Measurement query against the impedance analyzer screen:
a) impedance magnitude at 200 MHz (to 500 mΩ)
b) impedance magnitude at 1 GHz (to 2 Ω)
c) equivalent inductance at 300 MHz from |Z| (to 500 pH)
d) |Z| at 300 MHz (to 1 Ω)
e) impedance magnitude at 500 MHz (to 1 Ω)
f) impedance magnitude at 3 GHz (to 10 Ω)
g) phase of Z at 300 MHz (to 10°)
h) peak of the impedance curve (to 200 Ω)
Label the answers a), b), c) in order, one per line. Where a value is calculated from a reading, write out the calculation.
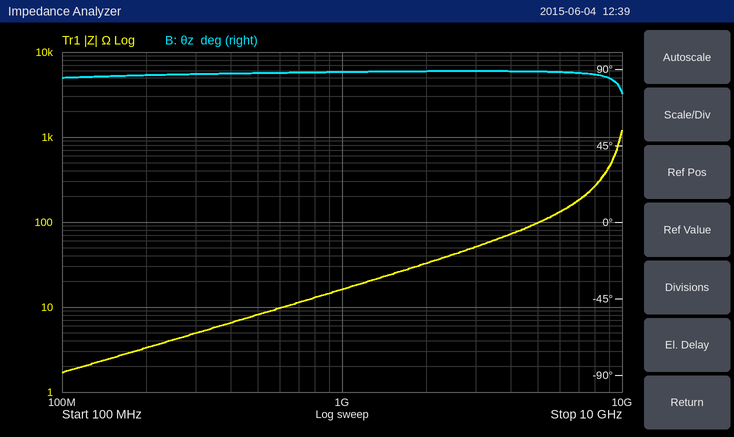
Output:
a) 3.5 Ω
b) 16 Ω
c) L = 5 Ω/(2π × 300 MHz) ≈ 2.65 nH, so 2.5 nH to the nearest 500 pH
d) 5 Ω
e) 8 Ω
f) 50 Ω
g) 90°
h) 1.2 kΩ
